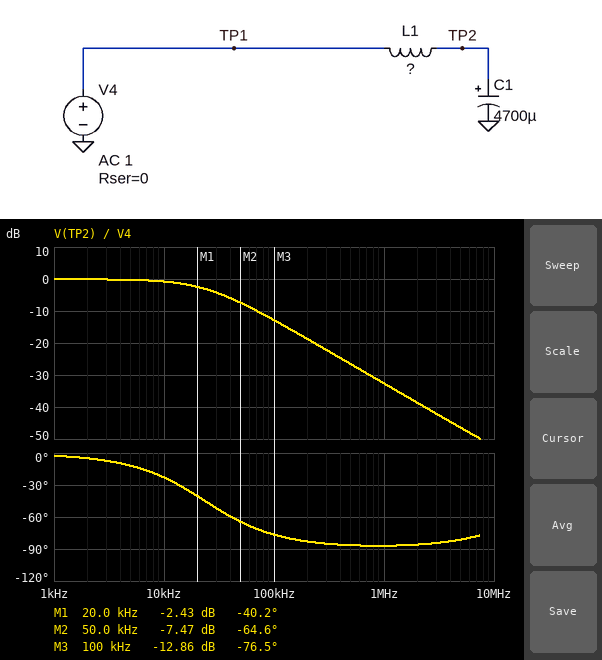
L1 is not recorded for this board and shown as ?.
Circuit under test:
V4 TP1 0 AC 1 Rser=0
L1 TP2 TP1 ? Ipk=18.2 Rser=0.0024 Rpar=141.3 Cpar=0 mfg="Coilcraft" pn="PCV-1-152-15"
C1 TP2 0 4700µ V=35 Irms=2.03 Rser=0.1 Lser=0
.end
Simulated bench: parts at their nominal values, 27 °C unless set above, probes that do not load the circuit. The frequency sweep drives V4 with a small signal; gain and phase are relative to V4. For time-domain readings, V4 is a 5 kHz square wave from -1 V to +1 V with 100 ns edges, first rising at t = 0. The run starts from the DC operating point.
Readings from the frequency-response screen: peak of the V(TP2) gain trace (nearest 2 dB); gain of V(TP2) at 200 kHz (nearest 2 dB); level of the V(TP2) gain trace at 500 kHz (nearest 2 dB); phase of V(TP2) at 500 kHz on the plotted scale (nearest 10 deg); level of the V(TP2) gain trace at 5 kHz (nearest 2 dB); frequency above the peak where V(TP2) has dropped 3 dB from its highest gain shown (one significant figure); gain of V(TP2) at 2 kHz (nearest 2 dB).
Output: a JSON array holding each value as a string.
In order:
["0 dB", "-18 dB", "-26 dB", "-90 deg", "0 dB", "20 kHz", "0 dB"]
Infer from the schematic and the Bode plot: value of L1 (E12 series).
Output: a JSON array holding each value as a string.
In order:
["680 nH"]
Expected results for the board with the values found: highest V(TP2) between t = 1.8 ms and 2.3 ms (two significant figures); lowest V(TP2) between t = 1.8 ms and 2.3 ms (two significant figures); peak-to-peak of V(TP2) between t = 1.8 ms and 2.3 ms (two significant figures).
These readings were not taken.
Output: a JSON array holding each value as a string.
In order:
["990 mV", "-990 mV", "2.0 V"]
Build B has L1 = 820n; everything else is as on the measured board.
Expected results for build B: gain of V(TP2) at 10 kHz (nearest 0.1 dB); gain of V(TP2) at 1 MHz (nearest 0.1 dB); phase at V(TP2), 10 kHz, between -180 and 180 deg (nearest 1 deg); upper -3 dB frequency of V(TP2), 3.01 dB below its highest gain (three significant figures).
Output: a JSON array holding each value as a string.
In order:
["-1.1 dB", "-34.2 dB", "-27 deg", "19.3 kHz"]
